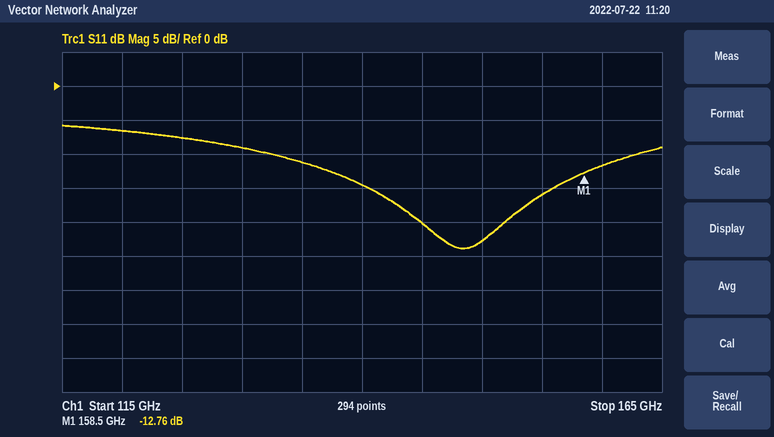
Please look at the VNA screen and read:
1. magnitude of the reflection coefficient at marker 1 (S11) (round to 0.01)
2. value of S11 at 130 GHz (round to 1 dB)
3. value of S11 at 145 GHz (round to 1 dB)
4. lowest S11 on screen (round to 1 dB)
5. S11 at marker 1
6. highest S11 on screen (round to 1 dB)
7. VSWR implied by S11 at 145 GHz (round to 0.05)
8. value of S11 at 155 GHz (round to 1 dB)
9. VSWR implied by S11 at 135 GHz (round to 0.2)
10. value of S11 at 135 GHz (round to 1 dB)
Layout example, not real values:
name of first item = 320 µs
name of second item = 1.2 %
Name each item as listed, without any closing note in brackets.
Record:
magnitude of the reflection coefficient at marker 1 (S11) = 0.23
value of S11 at 130 GHz = -9 dB
value of S11 at 145 GHz = -20 dB
lowest S11 on screen = -24 dB
S11 at marker 1 = -12.76 dB
highest S11 on screen = -6 dB
VSWR implied by S11 at 145 GHz = 1.20
value of S11 at 155 GHz = -16 dB
VSWR implied by S11 at 135 GHz = 1.8
value of S11 at 135 GHz = -11 dB
